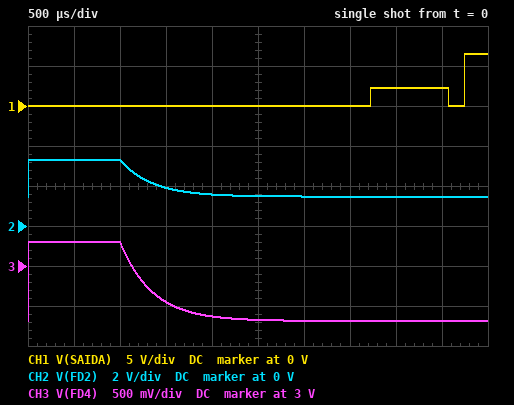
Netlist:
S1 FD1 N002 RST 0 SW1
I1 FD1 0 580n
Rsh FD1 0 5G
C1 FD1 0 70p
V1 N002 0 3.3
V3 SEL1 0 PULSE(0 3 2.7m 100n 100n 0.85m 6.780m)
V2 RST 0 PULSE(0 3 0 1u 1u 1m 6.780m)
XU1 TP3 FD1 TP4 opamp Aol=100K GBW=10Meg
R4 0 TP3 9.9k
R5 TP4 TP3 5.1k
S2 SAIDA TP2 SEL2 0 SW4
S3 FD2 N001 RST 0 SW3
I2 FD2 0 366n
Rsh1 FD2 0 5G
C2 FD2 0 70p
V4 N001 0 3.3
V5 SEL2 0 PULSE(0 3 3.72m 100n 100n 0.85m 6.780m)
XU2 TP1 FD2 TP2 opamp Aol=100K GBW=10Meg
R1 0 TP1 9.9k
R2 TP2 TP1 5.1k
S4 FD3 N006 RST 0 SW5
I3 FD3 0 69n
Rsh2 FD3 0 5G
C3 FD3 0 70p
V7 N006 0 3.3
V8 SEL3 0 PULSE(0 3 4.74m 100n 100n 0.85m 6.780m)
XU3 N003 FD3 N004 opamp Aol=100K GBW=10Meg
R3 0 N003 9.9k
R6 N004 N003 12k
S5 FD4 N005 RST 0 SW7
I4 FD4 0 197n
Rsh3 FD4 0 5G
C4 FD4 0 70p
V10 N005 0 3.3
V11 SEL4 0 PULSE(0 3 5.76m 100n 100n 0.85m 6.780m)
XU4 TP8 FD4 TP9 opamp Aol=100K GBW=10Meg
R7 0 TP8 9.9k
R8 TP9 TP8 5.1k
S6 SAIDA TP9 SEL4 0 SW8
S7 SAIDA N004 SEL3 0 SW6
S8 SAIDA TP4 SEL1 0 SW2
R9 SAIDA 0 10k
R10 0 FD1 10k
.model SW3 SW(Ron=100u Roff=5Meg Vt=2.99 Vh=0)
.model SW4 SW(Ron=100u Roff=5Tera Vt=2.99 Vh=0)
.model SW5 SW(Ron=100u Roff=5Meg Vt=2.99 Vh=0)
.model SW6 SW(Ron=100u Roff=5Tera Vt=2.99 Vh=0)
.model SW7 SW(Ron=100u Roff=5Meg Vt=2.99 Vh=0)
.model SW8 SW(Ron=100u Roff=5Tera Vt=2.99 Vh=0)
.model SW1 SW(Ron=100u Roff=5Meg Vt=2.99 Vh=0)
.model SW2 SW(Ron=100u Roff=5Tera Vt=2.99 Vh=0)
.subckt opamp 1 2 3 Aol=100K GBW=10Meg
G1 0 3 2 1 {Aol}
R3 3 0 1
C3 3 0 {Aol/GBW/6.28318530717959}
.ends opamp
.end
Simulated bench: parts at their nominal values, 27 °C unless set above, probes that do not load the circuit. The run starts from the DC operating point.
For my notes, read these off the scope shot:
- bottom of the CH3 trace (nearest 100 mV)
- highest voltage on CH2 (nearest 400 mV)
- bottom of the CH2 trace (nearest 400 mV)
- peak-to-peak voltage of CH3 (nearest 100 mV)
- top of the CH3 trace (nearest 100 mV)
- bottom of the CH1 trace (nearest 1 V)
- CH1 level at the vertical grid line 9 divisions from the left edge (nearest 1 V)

2.3 V
3.2 V
1.6 V
1.0 V
3.3 V
0 V
2 V
